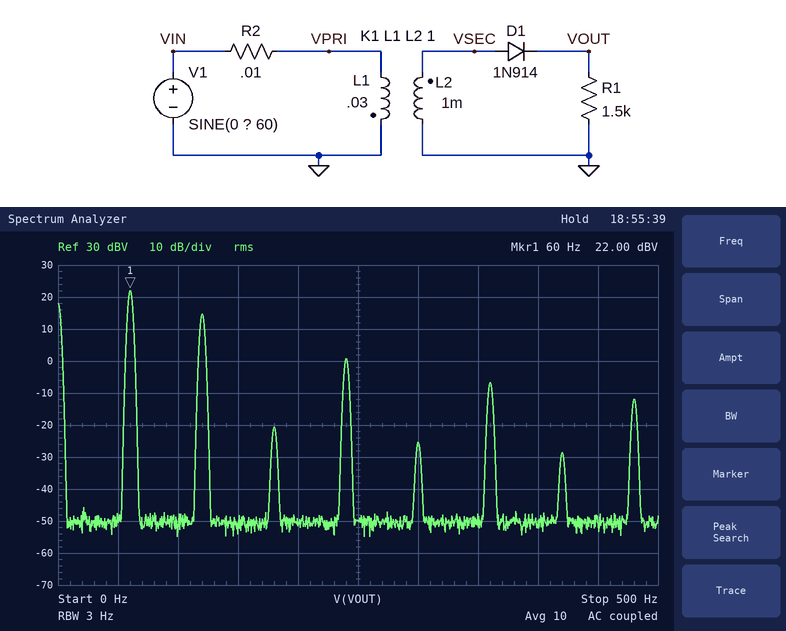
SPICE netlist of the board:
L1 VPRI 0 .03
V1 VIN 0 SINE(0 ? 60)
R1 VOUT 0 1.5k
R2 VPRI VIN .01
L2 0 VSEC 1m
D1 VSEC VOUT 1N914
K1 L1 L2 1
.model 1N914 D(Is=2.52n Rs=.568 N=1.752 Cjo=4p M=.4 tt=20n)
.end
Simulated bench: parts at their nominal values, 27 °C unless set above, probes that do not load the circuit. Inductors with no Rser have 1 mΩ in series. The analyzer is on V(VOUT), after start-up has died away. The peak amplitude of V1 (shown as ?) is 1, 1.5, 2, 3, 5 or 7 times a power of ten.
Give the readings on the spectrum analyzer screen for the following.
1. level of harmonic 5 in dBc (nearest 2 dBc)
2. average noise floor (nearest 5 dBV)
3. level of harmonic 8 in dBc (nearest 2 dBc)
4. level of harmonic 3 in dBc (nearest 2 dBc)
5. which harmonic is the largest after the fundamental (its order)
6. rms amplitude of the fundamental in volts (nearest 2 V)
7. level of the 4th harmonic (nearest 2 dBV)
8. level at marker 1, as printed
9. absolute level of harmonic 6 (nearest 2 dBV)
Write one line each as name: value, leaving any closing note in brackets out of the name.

level of harmonic 5 in dBc: -48 dBc
average noise floor: -50 dBV
level of harmonic 8 in dBc: -34 dBc
level of harmonic 3 in dBc: -42 dBc
which harmonic is the largest after the fundamental: 2
rms amplitude of the fundamental in volts: 12 V
level of the 4th harmonic: 0 dBV
level at marker 1, as printed: 22.00 dBV
absolute level of harmonic 6: -6 dBV
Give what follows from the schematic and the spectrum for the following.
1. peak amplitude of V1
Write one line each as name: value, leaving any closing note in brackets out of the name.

peak amplitude of V1: 200 V
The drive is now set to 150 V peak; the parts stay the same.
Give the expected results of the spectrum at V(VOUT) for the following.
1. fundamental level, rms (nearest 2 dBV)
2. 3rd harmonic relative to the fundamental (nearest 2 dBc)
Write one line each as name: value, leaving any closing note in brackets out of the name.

fundamental level, rms: 20 dBV
3rd harmonic relative to the fundamental: -40 dBc
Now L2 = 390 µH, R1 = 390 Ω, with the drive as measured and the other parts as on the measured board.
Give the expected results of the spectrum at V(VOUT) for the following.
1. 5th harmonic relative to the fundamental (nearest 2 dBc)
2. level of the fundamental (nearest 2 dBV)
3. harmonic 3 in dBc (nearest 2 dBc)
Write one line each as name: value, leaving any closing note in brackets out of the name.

5th harmonic relative to the fundamental: -42 dBc
level of the fundamental: 18 dBV
harmonic 3 in dBc: -38 dBc
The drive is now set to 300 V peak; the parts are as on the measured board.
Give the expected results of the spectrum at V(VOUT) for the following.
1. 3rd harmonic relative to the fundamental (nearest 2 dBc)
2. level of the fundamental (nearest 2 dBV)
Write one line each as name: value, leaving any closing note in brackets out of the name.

3rd harmonic relative to the fundamental: -46 dBc
level of the fundamental: 26 dBV
